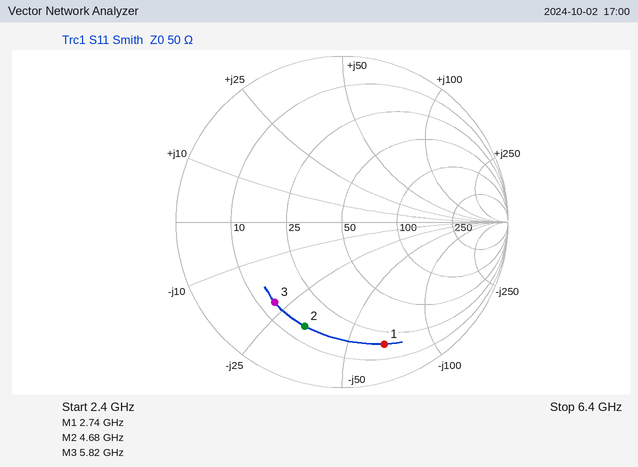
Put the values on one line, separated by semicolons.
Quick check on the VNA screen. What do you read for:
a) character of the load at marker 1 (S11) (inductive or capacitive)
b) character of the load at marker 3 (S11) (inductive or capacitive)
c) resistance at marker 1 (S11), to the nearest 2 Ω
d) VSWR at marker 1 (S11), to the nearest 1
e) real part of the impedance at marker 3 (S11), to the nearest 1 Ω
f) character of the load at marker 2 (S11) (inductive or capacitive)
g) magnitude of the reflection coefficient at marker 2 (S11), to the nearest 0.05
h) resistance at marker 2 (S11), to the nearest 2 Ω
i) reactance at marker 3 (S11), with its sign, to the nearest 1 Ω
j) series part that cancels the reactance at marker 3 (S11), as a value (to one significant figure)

capacitive; capacitive; 18 Ω; 8; 14 Ω; capacitive; 0.65; 14 Ω; -22 Ω; 600 pH
